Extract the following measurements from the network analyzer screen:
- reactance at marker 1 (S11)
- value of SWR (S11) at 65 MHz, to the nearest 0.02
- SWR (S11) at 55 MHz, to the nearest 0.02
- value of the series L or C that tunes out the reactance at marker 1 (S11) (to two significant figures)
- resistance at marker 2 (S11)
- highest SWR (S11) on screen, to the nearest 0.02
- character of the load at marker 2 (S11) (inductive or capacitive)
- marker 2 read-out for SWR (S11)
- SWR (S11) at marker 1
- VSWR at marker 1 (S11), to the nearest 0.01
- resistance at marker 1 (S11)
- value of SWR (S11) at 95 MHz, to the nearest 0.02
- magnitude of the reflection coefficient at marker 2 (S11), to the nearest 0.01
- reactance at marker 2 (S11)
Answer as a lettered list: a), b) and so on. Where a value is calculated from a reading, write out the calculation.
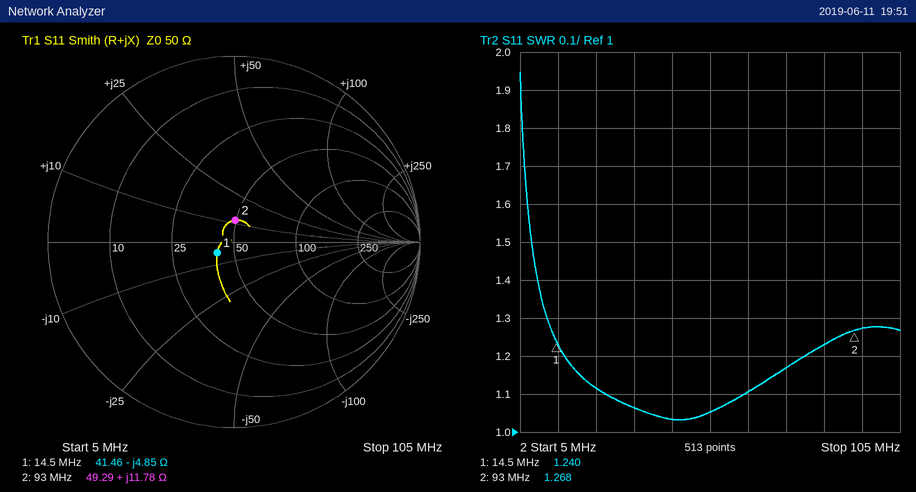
a) -4.85 Ω
b) 1.10
c) 1.06
d) L = 4.85 Ω/(2π × 14.5 MHz) ≈ 53 nH
e) 49.29 Ω
f) 1.94
g) inductive
h) 1.268
i) 1.240
j) 1.24
k) 41.46 Ω
l) 1.28
m) 0.12
n) +11.78 Ω
